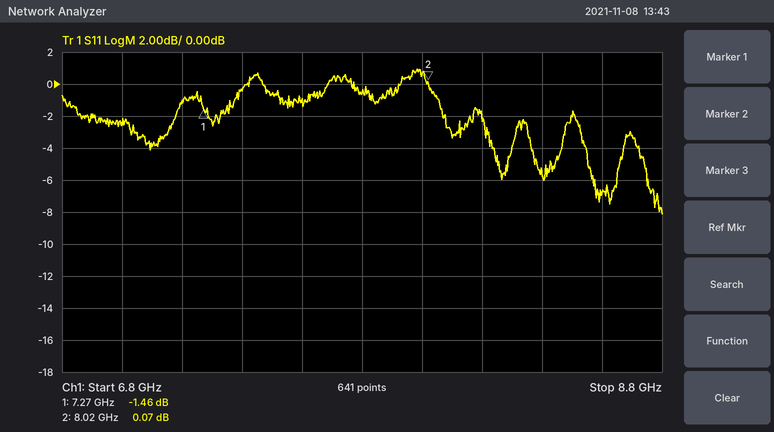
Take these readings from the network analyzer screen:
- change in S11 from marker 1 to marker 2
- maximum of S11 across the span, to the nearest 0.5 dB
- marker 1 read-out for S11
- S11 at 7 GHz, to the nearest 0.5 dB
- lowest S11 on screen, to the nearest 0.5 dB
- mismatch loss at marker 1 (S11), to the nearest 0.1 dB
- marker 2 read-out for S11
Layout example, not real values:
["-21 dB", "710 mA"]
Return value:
["1.53 dB", "1.0 dB", "-1.46 dB", "-2.5 dB", "-8.0 dB", "5.4 dB", "0.07 dB"]
